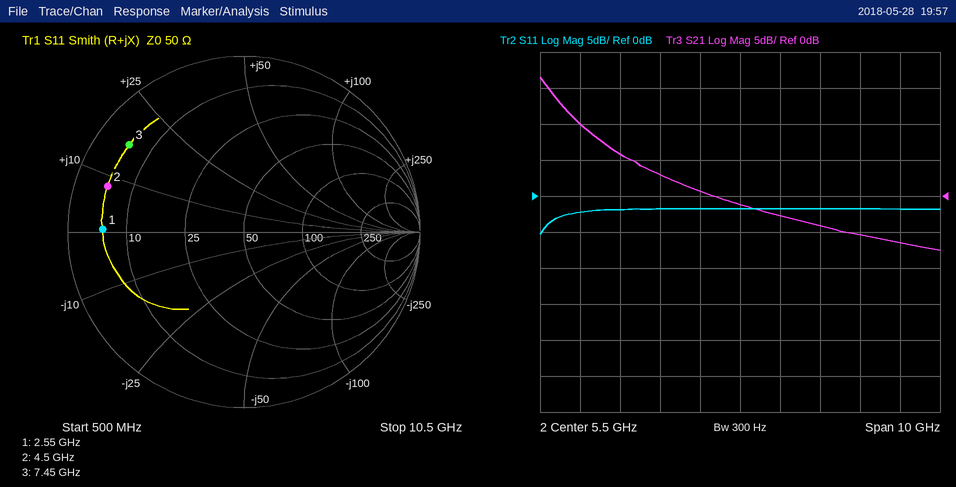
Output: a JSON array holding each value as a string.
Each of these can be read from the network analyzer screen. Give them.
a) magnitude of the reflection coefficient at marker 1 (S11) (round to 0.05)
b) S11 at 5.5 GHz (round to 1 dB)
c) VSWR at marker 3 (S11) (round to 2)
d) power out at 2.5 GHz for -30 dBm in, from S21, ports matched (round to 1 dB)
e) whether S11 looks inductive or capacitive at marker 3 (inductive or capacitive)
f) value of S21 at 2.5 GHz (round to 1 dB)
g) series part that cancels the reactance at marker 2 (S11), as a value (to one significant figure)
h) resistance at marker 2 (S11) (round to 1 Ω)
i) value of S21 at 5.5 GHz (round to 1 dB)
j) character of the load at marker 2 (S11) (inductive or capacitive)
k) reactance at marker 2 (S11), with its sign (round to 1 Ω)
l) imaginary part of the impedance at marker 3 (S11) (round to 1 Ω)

["0.80", "-2 dB", "10", "-24 dBm", "inductive", "6 dB", "4 pF", "5 Ω", "-1 dB", "inductive", "+8 Ω", "+17 Ω"]
